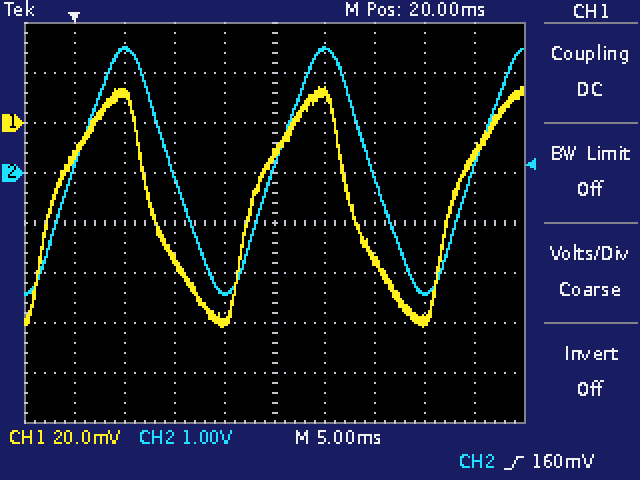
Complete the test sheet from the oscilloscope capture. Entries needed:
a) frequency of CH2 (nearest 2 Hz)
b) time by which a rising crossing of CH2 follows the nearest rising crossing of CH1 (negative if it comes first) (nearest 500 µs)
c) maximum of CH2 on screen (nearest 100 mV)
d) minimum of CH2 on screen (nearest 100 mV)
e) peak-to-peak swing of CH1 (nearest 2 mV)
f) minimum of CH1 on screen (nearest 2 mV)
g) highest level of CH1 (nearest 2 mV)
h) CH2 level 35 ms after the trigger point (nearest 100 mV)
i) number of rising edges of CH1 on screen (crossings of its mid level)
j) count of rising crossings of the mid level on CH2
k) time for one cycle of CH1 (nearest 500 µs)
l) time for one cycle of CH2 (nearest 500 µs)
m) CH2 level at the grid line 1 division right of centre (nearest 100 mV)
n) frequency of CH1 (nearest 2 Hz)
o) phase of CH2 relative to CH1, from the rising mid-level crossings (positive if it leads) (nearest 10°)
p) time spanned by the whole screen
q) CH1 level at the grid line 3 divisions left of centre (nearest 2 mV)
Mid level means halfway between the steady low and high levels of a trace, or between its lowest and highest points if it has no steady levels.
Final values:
50 Hz
+2.0 ms
2.5 V
-2.4 V
96 mV
-82 mV
14 mV
-2.4 V
3
3
20.0 ms
20.0 ms
2.5 V
50 Hz
-40°
50 ms
12 mV
